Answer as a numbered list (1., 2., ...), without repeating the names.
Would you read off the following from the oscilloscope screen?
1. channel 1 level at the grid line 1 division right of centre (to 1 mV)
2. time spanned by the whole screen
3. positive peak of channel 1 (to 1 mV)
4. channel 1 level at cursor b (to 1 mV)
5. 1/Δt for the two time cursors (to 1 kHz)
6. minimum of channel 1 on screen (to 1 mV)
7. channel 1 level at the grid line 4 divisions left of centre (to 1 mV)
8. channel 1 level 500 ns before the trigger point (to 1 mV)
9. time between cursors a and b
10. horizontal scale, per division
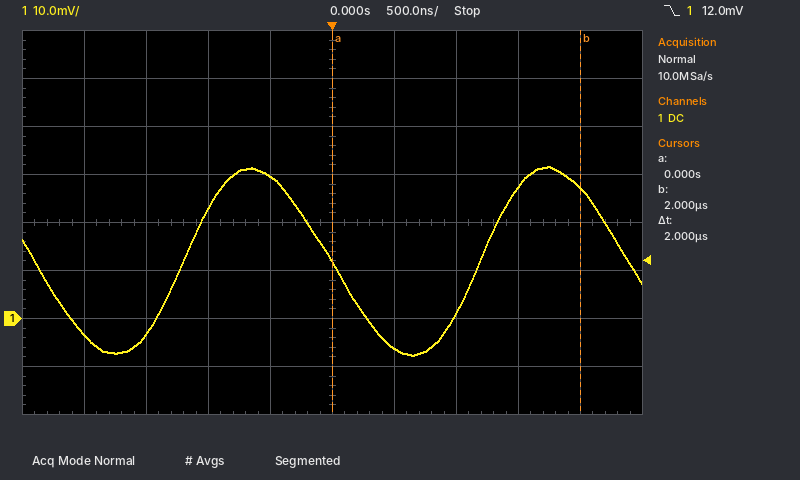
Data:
1. -6 mV
2. 5 µs
3. 32 mV
4. 27 mV
5. 500 kHz
6. -8 mV
7. -3 mV
8. 30 mV
9. 2 µs
10. 500 ns
